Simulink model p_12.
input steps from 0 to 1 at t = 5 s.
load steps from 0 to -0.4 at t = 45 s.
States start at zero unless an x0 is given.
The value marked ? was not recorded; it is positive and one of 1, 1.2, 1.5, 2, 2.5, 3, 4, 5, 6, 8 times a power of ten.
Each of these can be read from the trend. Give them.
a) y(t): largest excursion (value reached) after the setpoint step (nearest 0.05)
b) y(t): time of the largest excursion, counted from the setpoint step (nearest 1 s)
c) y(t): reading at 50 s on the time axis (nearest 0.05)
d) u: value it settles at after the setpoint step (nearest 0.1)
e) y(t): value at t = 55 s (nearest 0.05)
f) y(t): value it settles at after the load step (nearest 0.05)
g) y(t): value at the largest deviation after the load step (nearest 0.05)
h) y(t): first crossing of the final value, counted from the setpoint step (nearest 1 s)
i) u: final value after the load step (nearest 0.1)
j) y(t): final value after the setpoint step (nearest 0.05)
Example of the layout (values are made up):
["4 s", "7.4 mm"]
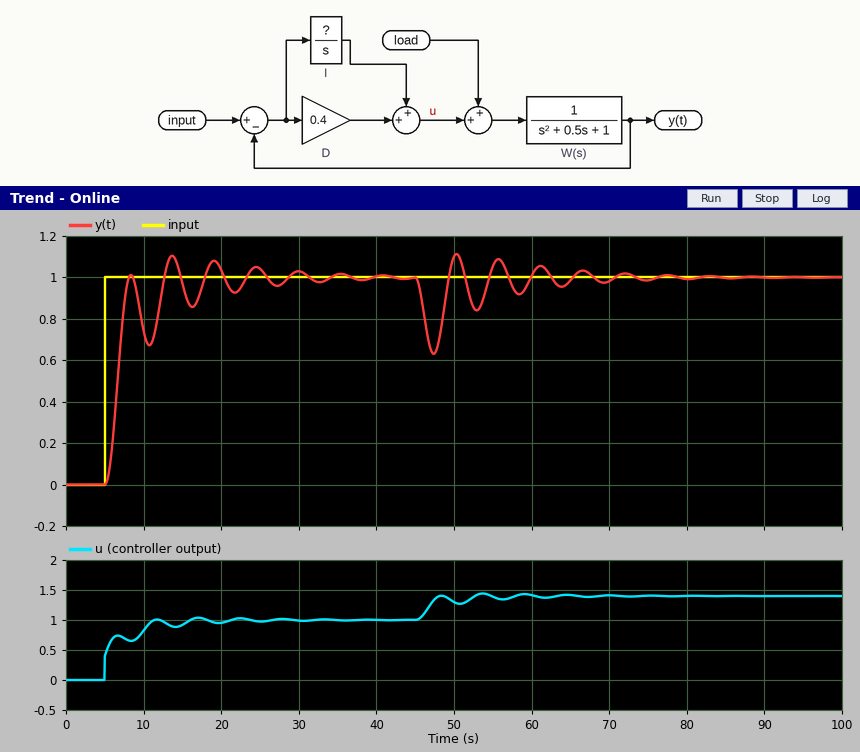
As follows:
["1.10", "9 s", "1.10", "1.0", "1.05", "1.00", "0.65", "3 s", "1.4", "1.00"]
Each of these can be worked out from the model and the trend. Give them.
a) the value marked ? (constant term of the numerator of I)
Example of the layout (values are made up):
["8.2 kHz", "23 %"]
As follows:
["0.4"]
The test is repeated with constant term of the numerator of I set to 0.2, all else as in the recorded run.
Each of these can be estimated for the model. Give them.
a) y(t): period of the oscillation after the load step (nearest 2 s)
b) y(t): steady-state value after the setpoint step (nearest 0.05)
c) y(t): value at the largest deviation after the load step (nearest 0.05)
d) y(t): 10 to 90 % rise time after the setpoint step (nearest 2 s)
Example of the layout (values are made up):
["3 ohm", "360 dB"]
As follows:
["6 s", "1.00", "0.60", "12 s"]
